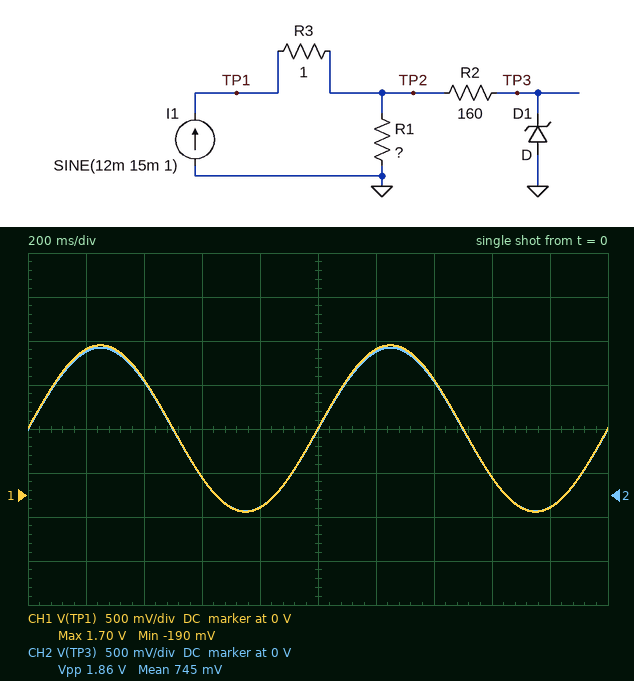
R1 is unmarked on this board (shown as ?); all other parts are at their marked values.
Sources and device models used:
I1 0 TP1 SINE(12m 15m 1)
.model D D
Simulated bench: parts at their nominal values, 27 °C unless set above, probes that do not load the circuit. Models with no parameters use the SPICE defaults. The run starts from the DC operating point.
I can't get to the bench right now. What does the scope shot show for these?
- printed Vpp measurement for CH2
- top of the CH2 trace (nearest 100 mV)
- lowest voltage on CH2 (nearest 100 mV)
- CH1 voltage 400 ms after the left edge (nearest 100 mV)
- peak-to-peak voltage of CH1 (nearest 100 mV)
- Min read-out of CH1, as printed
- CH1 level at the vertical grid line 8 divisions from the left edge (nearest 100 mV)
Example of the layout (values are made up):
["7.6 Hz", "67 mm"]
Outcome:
["1.86 V", "1.7 V", "-200 mV", "1.3 V", "1.9 V", "-190 mV", "200 mV"]
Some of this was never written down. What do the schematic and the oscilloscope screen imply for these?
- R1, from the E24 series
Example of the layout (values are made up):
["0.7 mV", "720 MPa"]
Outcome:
["62 Ω"]
